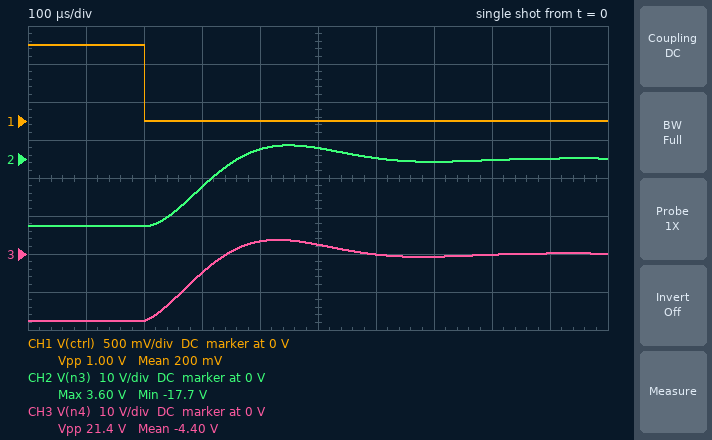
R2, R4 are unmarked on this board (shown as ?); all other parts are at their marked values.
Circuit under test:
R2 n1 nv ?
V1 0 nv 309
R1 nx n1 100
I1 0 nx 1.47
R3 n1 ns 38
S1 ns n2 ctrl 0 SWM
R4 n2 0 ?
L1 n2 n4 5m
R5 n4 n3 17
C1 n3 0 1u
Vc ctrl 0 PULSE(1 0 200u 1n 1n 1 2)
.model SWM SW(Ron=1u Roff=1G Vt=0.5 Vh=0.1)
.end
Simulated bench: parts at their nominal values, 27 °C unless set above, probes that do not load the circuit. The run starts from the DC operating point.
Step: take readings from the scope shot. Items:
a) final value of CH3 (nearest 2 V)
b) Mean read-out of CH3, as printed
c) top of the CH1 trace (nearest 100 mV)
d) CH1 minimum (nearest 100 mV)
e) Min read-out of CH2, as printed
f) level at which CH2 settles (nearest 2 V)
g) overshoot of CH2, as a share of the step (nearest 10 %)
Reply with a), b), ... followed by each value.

a) 0 V
b) -4.40 V
c) 1.0 V
d) 0 V
e) -17.7 V
f) 0 V
g) 20 %
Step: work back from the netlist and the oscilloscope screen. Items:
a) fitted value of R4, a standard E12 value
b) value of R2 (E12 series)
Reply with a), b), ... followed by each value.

a) 47 Ω
b) 150 Ω
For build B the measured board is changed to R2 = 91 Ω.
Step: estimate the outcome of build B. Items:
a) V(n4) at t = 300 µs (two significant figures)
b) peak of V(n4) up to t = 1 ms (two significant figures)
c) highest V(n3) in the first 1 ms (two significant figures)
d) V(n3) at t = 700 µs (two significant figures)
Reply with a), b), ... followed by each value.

a) -13 V
b) 9.8 V
c) 9.5 V
d) -1.9 V
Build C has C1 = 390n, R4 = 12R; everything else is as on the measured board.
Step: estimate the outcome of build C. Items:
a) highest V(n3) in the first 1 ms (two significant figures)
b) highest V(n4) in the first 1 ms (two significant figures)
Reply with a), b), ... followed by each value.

a) 3.5 V
b) 3.6 V
